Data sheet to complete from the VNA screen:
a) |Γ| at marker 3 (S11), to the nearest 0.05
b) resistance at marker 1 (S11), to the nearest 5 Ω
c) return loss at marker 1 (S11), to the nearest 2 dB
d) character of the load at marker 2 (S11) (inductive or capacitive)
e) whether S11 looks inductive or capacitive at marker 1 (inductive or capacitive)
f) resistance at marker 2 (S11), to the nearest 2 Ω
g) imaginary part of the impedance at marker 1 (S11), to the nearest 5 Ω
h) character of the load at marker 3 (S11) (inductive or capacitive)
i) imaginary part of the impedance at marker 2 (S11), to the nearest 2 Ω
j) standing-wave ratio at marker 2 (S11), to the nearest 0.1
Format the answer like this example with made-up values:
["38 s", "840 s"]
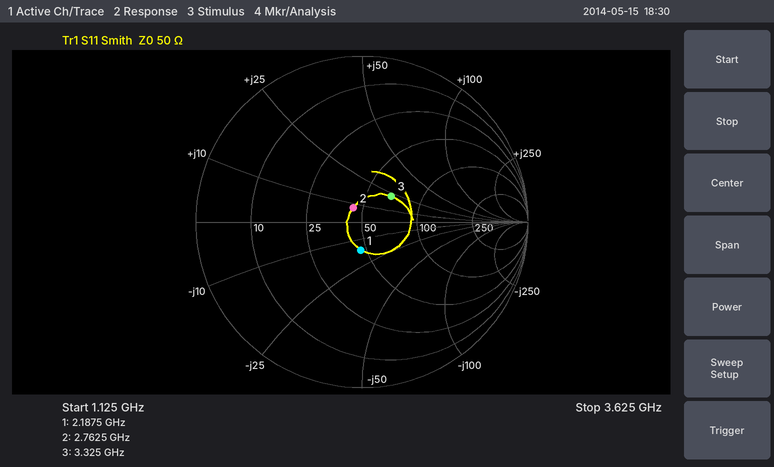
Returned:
["0.25", "45 Ω", "16 dB", "inductive", "capacitive", "44 Ω", "-15 Ω", "inductive", "+8 Ω", "1.2"]
